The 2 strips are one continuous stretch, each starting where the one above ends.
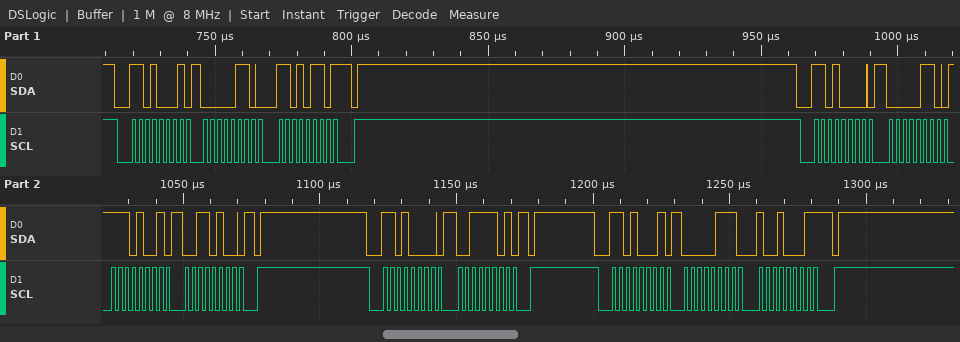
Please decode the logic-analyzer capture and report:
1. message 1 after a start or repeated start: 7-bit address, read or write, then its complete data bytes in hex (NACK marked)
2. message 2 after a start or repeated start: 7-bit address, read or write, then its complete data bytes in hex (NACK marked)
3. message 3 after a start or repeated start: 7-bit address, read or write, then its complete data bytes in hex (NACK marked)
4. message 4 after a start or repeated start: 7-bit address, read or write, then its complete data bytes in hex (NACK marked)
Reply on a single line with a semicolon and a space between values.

0x68 read: 06 D6 NACK; 0x68 write: 06 E9 34; 0x68 write: 3D; 0x68 read: 07 91 NACK
